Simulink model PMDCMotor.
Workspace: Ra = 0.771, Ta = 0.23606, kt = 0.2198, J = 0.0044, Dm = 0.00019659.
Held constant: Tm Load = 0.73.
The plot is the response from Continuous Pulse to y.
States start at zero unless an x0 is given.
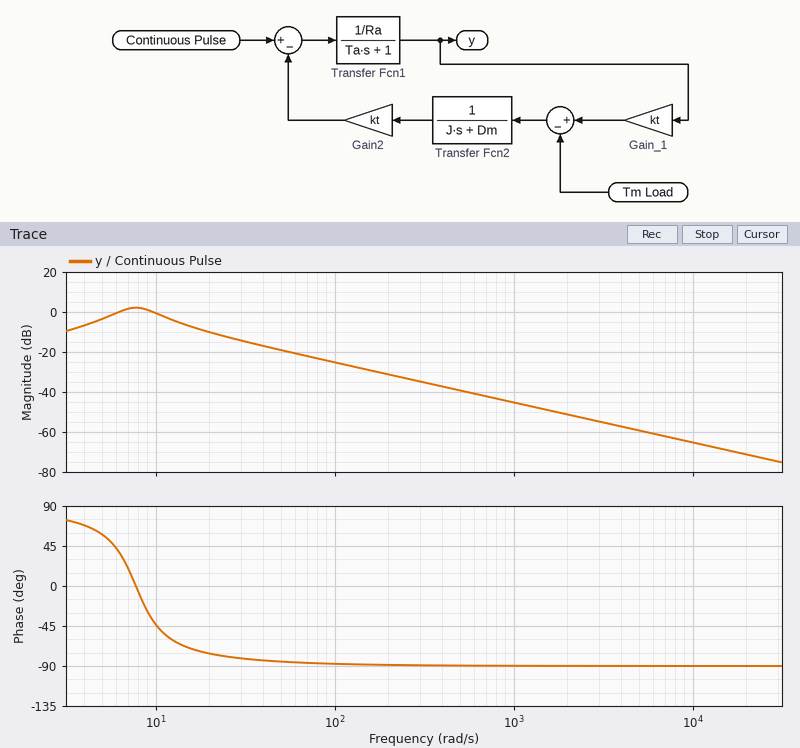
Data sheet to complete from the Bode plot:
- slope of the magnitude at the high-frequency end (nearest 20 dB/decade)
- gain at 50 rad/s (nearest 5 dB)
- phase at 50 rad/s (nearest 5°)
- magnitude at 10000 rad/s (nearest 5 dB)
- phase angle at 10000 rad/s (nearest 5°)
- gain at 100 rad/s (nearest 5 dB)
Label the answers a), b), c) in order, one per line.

a) -20 dB/decade
b) -20 dB
c) -85°
d) -65 dB
e) -90°
f) -25 dB
